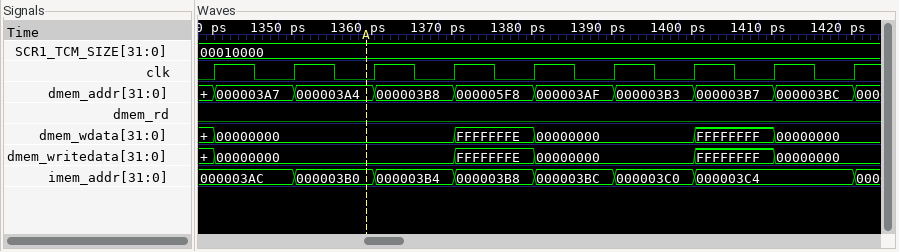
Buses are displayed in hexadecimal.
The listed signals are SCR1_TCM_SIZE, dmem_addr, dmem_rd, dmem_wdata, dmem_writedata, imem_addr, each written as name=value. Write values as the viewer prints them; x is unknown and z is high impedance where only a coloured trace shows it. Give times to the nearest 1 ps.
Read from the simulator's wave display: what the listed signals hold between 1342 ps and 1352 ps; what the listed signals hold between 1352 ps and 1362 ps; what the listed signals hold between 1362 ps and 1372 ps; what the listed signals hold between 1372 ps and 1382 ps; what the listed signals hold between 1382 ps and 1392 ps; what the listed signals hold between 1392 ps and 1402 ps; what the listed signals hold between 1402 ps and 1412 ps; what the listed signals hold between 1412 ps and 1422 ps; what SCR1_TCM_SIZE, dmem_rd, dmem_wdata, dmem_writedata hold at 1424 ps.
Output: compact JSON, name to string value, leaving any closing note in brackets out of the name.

{"what the listed signals hold between 1342 ps and 1352 ps": "SCR1_TCM_SIZE=00010000, dmem_addr=000003A7, dmem_rd=0, dmem_wdata=00000000, dmem_writedata=00000000, imem_addr=000003AC", "what the listed signals hold between 1352 ps and 1362 ps": "SCR1_TCM_SIZE=00010000, dmem_addr=000003A4, dmem_rd=0, dmem_wdata=00000000, dmem_writedata=00000000, imem_addr=000003B0", "what the listed signals hold between 1362 ps and 1372 ps": "SCR1_TCM_SIZE=00010000, dmem_addr=000003B8, dmem_rd=0, dmem_wdata=00000000, dmem_writedata=00000000, imem_addr=000003B4", "what the listed signals hold between 1372 ps and 1382 ps": "SCR1_TCM_SIZE=00010000, dmem_addr=000005F8, dmem_rd=0, dmem_wdata=FFFFFFFE, dmem_writedata=FFFFFFFE, imem_addr=000003B8", "what the listed signals hold between 1382 ps and 1392 ps": "SCR1_TCM_SIZE=00010000, dmem_addr=000003AF, dmem_rd=0, dmem_wdata=00000000, dmem_writedata=00000000, imem_addr=000003BC", "what the listed signals hold between 1392 ps and 1402 ps": "SCR1_TCM_SIZE=00010000, dmem_addr=000003B3, dmem_rd=0, dmem_wdata=00000000, dmem_writedata=00000000, imem_addr=000003C0", "what the listed signals hold between 1402 ps and 1412 ps": "SCR1_TCM_SIZE=00010000, dmem_addr=000003B7, dmem_rd=0, dmem_wdata=FFFFFFFF, dmem_writedata=FFFFFFFF, imem_addr=000003C4", "what the listed signals hold between 1412 ps and 1422 ps": "SCR1_TCM_SIZE=00010000, dmem_addr=000003BC, dmem_rd=0, dmem_wdata=00000000, dmem_writedata=00000000, imem_addr=000003C4", "what SCR1_TCM_SIZE, dmem_rd, dmem_wdata, dmem_writedata hold at 1424 ps": "SCR1_TCM_SIZE=00010000, dmem_rd=0, dmem_wdata=00000000, dmem_writedata=00000000"}
